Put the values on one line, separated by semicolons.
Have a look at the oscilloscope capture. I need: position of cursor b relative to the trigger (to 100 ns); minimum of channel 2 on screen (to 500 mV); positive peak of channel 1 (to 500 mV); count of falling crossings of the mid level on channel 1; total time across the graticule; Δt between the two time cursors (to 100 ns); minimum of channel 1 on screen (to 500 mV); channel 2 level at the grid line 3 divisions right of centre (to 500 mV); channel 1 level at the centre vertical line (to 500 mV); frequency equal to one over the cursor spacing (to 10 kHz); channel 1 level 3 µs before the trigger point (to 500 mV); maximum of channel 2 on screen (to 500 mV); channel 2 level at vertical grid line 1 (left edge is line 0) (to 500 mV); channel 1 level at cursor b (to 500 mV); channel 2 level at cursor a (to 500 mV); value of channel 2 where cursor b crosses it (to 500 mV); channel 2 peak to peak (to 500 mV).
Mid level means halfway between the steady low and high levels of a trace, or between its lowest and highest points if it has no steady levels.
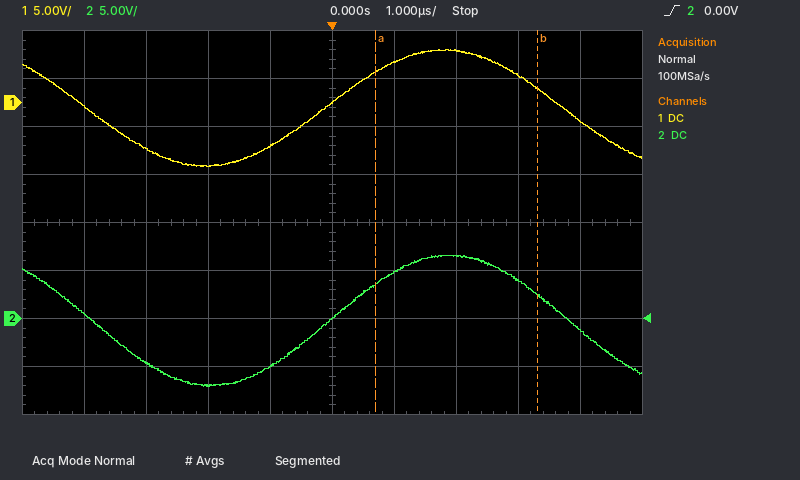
+3.3 µs; -7.0 V; 5.5 V; 2; 10 µs; 2.6 µs; -6.5 V; 4.0 V; 0.0 V; 380 kHz; -5.0 V; 6.5 V; 500 mV; 1.5 V; 3.5 V; 2.5 V; 13.5 V
